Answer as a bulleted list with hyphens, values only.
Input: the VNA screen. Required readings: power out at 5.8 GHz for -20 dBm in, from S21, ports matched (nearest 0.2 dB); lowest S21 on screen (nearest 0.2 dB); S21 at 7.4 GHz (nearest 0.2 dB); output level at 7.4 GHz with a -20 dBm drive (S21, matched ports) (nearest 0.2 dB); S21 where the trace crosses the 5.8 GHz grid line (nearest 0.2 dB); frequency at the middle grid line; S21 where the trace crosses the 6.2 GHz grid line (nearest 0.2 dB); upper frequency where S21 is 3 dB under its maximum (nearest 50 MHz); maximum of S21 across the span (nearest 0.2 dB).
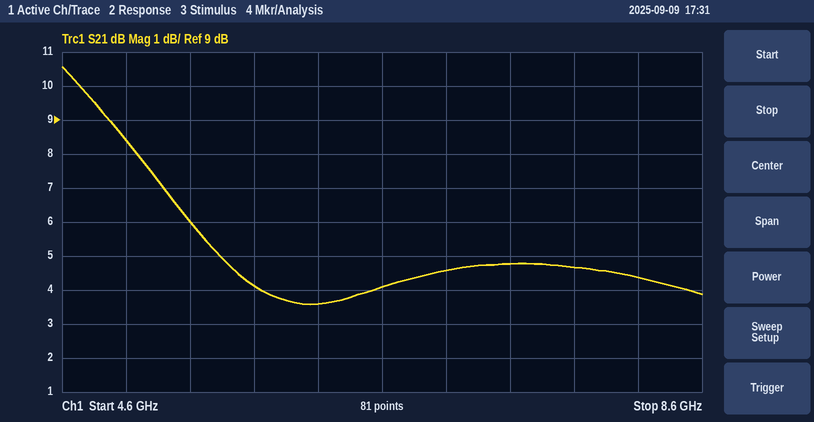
- -15.8 dBm
- 3.6 dB
- 4.8 dB
- -15.2 dBm
- 4.2 dB
- 6.6 GHz
- 3.6 dB
- 5.15 GHz
- 10.6 dB
